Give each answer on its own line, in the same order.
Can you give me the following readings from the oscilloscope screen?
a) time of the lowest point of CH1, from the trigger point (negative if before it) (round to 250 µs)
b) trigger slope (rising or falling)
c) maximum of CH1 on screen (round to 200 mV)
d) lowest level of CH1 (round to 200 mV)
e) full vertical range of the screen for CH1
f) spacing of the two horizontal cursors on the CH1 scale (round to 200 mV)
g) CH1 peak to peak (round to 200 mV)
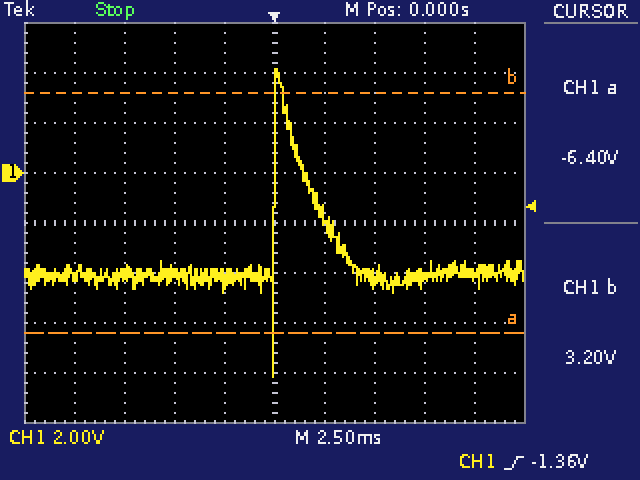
0.00 ms
rising
4.2 V
-8.2 V
16 V
9.6 V
12.4 V
